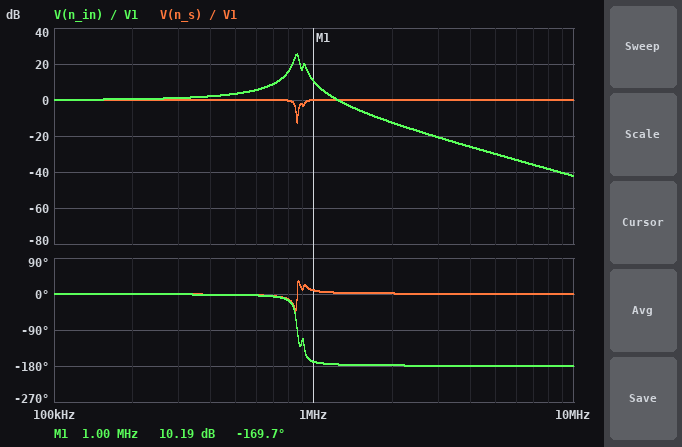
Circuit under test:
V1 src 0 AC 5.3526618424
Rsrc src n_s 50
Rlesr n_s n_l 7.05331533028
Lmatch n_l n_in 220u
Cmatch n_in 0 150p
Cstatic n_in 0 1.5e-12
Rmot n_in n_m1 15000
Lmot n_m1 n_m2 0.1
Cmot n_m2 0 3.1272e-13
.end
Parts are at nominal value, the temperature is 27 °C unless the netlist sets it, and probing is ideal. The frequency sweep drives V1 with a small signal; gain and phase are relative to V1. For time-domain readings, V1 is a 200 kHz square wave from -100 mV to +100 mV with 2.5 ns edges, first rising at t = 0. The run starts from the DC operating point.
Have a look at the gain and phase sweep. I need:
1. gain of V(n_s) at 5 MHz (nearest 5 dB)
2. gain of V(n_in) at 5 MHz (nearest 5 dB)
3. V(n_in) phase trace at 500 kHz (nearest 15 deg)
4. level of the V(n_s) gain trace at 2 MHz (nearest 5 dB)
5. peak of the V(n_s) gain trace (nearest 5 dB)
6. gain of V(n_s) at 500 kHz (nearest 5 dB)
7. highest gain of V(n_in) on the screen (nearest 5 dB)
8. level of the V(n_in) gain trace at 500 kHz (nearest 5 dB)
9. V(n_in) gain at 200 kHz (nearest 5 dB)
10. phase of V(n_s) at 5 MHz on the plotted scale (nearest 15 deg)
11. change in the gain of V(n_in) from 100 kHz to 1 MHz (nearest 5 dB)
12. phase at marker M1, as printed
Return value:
0 dB
-30 dB
0 deg
0 dB
0 dB
0 dB
25 dB
5 dB
0 dB
0 deg
10 dB
-169.7 deg
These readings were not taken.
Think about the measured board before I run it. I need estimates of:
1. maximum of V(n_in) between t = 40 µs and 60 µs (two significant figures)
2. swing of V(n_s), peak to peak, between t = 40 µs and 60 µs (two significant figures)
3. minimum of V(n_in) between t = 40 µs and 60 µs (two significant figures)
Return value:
230 mV
210 mV
-230 mV
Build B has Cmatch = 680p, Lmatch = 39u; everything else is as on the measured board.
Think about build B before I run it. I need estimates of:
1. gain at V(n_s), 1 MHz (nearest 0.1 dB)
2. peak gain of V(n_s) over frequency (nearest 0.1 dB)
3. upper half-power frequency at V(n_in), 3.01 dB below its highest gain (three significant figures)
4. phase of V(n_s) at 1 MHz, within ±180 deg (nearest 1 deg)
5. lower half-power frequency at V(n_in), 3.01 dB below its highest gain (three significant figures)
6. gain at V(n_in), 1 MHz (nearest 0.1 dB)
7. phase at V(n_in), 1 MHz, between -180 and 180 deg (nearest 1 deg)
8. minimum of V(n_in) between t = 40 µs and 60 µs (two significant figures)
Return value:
-12.9 dB
0 dB
1.07 MHz
46 deg
836 kHz
12.1 dB
-101 deg
-260 mV
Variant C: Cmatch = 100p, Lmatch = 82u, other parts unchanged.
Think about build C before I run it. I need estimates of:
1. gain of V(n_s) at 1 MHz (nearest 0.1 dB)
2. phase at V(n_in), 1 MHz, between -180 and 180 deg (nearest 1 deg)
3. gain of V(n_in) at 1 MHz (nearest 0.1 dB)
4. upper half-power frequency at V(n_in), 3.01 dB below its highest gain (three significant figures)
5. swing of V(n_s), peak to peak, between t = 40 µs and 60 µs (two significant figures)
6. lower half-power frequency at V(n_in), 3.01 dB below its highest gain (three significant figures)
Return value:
0 dB
-3 deg
3.4 dB
1.80 MHz
220 mV
1.69 MHz
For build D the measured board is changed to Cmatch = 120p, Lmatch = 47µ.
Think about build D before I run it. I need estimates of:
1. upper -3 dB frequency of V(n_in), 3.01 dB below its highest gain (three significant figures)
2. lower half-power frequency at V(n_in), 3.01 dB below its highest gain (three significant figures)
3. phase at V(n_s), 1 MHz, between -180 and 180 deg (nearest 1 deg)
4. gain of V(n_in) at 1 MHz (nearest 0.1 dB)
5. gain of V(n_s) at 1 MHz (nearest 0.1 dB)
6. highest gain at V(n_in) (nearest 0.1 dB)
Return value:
2.20 MHz
2.00 MHz
-3 deg
2.2 dB
0 dB
20.8 dB
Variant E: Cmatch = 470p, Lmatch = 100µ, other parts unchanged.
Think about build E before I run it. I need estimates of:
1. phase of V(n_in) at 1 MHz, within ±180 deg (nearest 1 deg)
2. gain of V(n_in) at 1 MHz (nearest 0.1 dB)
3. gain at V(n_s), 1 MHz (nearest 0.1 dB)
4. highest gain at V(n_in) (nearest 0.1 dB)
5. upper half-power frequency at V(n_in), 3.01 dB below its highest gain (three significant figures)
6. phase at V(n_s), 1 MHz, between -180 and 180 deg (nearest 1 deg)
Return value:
-169 deg
1.2 dB
-0.2 dB
18.1 dB
773 kHz
10 deg
